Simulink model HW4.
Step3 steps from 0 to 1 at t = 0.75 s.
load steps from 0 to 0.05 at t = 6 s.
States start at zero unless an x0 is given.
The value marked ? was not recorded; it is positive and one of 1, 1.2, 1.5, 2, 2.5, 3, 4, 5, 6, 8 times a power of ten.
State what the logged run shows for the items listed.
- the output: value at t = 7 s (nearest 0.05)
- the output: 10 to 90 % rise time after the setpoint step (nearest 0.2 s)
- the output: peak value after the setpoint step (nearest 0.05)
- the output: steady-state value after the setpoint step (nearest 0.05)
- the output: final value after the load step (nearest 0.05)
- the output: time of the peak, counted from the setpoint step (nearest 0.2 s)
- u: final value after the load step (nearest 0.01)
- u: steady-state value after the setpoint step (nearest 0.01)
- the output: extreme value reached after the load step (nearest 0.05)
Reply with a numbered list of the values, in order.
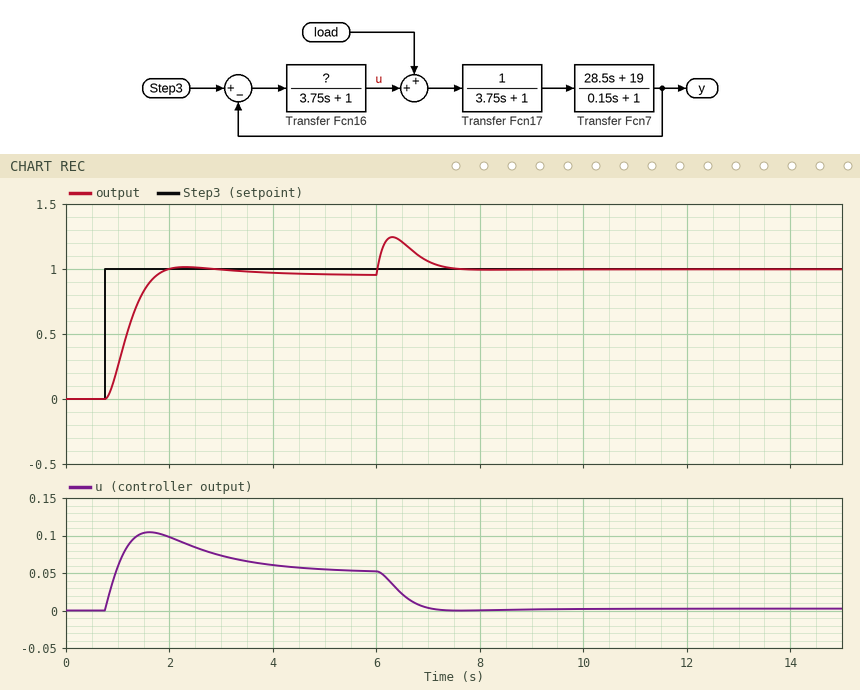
1. 1.05
2. 0.6 s
3. 1.00
4. 0.95
5. 1.00
6. 1.6 s
7. 0.00
8. 0.05
9. 1.25
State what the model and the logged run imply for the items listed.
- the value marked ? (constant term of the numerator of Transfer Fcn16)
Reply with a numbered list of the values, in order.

1. 1
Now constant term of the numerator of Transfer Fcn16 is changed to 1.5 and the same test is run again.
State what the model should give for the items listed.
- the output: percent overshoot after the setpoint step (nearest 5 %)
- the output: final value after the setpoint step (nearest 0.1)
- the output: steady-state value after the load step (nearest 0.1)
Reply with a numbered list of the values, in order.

1. 10 %
2. 1.0
3. 1.0
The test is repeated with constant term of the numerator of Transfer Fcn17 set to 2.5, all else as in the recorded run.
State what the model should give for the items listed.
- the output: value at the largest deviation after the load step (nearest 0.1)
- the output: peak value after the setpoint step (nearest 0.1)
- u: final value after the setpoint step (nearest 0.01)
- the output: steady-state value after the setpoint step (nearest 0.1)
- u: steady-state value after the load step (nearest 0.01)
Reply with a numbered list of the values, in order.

1. 1.6
2. 1.1
3. 0.02
4. 1.0
5. -0.03
